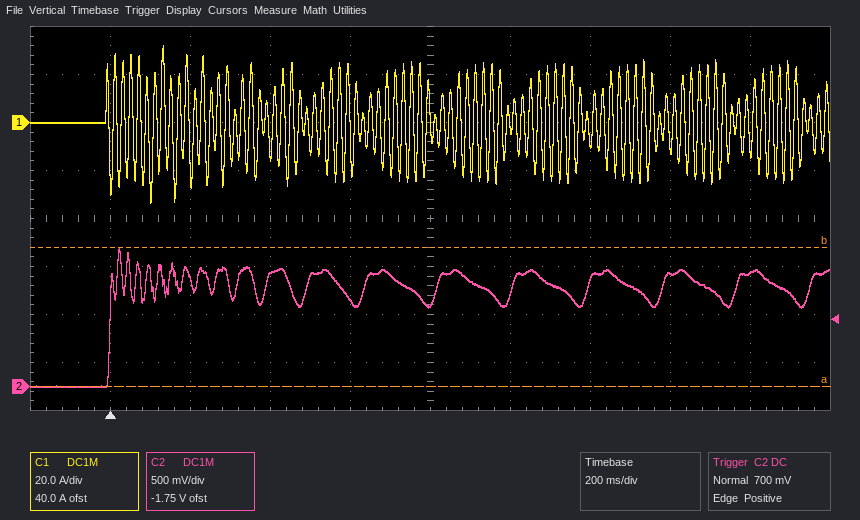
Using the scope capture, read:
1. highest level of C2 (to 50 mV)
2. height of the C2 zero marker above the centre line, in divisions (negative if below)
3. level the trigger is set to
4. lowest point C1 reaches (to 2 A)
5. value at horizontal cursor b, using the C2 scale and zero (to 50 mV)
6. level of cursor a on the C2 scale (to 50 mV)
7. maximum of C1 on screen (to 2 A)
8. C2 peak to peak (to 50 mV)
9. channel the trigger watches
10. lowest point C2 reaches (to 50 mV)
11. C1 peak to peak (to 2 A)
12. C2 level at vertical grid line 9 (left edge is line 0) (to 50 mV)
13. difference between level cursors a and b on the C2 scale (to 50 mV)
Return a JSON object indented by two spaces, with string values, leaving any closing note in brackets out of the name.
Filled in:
{
  "highest level of C2": "1.45 V",
  "height of the C2 zero marker above the centre line, in divisions": "-3.5 div",
  "level the trigger is set to": "700 mV",
  "lowest point C1 reaches": "-34 A",
  "value at horizontal cursor b, using the C2 scale and zero": "1.45 V",
  "level of cursor a on the C2 scale": "0 mV",
  "maximum of C1 on screen": "32 A",
  "C2 peak to peak": "1.45 V",
  "channel the trigger watches": "C2",
  "lowest point C2 reaches": "0 mV",
  "C1 peak to peak": "66 A",
  "C2 level at vertical grid line 9 (left edge is line 0)": "1.20 V",
  "difference between level cursors a and b on the C2 scale": "1.45 V"
}
